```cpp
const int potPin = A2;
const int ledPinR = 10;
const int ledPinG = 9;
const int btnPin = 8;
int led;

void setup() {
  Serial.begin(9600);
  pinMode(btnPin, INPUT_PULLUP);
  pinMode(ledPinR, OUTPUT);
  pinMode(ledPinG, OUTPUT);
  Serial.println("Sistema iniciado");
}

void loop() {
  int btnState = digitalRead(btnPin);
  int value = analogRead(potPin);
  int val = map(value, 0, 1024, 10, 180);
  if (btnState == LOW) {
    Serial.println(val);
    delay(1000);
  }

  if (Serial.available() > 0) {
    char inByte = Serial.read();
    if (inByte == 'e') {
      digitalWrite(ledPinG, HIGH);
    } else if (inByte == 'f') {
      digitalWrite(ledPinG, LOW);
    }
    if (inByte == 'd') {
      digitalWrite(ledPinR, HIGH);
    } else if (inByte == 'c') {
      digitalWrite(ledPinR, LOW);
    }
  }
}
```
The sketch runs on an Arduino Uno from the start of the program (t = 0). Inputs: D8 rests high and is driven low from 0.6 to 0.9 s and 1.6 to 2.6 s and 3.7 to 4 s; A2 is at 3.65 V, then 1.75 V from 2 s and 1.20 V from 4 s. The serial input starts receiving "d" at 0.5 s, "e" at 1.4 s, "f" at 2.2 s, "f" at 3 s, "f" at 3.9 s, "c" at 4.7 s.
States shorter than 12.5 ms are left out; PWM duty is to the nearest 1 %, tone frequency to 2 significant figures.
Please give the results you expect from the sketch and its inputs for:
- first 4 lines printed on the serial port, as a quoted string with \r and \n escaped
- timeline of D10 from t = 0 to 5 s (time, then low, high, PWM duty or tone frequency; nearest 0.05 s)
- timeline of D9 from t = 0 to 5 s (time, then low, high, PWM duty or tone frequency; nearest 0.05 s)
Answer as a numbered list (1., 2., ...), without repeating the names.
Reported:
1. "Sistema iniciado\r\n134\r\n134\r\n69\r\n"
2. 0 s low; 0.5 s high; 4.7 s low
3. 0 s low; 1.6 s high; 2.6 s low
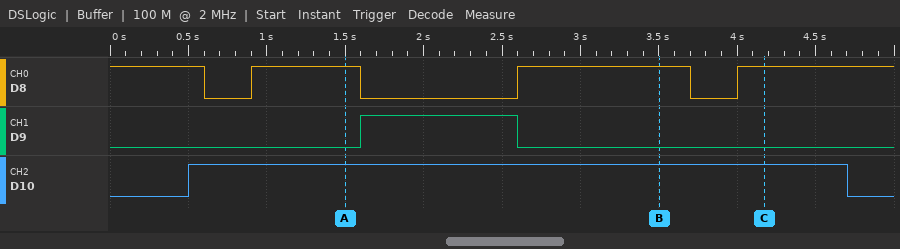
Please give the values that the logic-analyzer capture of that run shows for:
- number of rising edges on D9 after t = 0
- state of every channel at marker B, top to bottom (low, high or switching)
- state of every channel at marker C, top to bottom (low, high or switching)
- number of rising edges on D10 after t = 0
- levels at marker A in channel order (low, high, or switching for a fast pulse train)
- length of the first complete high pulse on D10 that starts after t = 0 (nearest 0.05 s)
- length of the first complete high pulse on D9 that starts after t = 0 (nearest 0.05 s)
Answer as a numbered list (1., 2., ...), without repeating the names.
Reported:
1. 1
2. D8 high, D9 low, D10 high
3. D8 high, D9 low, D10 high
4. 1
5. D8 high, D9 low, D10 high
6. 4.20 s
7. 1.00 s
